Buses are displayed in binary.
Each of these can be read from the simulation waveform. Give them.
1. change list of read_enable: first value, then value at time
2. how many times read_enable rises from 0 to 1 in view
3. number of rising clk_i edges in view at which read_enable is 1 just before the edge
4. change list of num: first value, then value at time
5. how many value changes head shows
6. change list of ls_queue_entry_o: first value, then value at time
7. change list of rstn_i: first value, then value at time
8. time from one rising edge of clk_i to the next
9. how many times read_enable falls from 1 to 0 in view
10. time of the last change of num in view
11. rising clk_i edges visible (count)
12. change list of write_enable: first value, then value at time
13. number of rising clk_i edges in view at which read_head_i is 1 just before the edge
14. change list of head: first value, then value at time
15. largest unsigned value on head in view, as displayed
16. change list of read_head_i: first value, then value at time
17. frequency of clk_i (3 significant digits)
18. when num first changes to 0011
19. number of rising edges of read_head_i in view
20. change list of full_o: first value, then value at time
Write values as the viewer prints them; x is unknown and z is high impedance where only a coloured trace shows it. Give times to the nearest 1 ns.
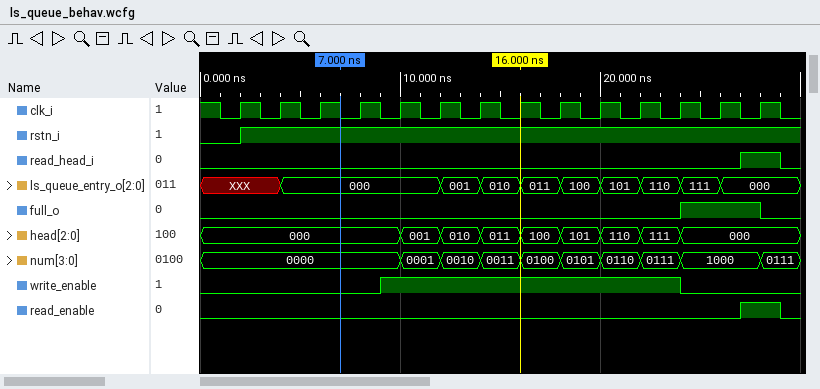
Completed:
0, 1 at 27 ns, 0 at 29 ns
1
1
0000, 0001 at 10 ns, 0010 at 12 ns, 0011 at 14 ns, 0100 at 16 ns, 0101 at 18 ns, 0110 at 20 ns, 0111 at 22 ns, 1000 at 24 ns, 0111 at 28 ns
8
XXX, 000 at 4 ns, 001 at 12 ns, 010 at 14 ns, 011 at 16 ns, 100 at 18 ns, 101 at 20 ns, 110 at 22 ns, 111 at 24 ns, 000 at 26 ns
0, 1 at 2 ns
2 ns
1
28 ns
14
0, 1 at 9 ns, 0 at 24 ns
1
000, 001 at 10 ns, 010 at 12 ns, 011 at 14 ns, 100 at 16 ns, 101 at 18 ns, 110 at 20 ns, 111 at 22 ns, 000 at 24 ns
111
0, 1 at 27 ns, 0 at 29 ns
500 MHz
14 ns
1
0, 1 at 24 ns, 0 at 28 ns
